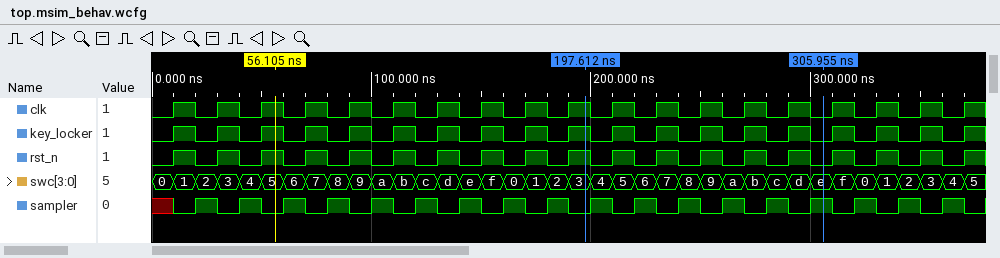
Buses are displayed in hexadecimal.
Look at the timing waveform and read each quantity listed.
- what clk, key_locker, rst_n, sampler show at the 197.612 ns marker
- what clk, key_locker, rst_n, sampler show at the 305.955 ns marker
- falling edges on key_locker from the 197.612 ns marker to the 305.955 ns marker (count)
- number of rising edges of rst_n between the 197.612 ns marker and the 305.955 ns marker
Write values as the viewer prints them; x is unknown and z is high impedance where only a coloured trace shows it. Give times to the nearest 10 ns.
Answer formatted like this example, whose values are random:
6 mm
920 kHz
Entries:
clk=1, key_locker=1, rst_n=1, sampler=0
clk=0, key_locker=0, rst_n=0, sampler=1
6
5
